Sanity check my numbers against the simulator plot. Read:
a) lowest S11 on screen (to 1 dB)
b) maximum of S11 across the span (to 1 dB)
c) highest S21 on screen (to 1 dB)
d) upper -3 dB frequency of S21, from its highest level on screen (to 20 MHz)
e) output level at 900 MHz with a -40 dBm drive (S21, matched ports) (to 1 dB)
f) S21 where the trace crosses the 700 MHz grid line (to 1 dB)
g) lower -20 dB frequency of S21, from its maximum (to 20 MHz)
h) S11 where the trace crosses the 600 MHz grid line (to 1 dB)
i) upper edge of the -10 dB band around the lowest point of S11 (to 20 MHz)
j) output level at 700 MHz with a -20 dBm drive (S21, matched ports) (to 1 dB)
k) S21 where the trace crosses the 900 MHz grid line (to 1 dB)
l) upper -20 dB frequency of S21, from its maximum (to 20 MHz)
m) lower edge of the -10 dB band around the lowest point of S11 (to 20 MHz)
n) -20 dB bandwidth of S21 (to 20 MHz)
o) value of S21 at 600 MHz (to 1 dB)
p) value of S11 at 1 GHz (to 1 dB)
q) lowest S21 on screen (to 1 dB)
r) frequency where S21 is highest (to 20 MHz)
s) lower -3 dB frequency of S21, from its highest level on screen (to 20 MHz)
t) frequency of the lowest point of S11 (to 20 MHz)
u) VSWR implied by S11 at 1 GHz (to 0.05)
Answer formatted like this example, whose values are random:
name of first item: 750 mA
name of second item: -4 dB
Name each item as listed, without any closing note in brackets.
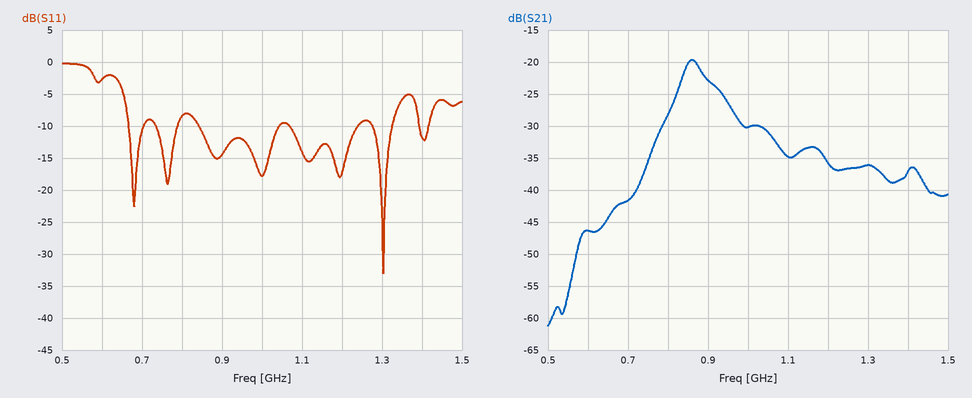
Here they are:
lowest S11 on screen: -33 dB
maximum of S11 across the span: 0 dB
highest S21 on screen: -20 dB
upper -3 dB frequency of S21, from its highest level on screen: 900 MHz
output level at 900 MHz with a -40 dBm drive (S21, matched ports): -63 dBm
S21 where the trace crosses the 700 MHz grid line: -42 dB
lower -20 dB frequency of S21, from its maximum: 720 MHz
S11 where the trace crosses the 600 MHz grid line: -3 dB
upper edge of the -10 dB band around the lowest point of S11: 1.32 GHz
output level at 700 MHz with a -20 dBm drive (S21, matched ports): -62 dBm
S21 where the trace crosses the 900 MHz grid line: -23 dB
upper -20 dB frequency of S21, from its maximum: 1.44 GHz
lower edge of the -10 dB band around the lowest point of S11: 1.28 GHz
-20 dB bandwidth of S21: 720 MHz
value of S21 at 600 MHz: -46 dB
value of S11 at 1 GHz: -18 dB
lowest S21 on screen: -61 dB
frequency where S21 is highest: 860 MHz
lower -3 dB frequency of S21, from its highest level on screen: 840 MHz
frequency of the lowest point of S11: 1.30 GHz
VSWR implied by S11 at 1 GHz: 1.30
